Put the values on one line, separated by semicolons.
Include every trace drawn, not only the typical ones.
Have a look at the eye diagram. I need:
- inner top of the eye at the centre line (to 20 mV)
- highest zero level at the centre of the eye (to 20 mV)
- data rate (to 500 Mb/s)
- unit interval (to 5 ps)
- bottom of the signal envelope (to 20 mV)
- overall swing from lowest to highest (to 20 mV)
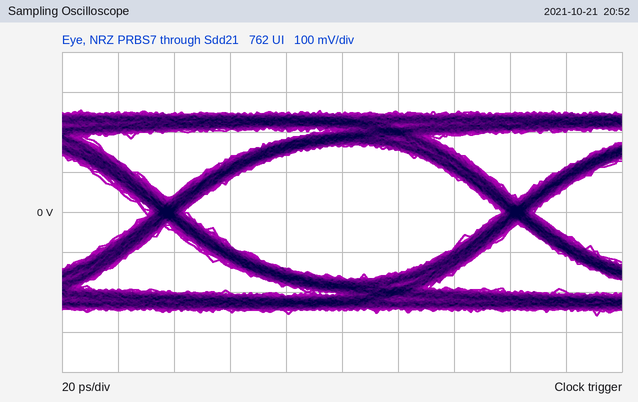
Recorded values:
160 mV; -160 mV; 8.0 Gb/s; 125 ps; -260 mV; 520 mV
